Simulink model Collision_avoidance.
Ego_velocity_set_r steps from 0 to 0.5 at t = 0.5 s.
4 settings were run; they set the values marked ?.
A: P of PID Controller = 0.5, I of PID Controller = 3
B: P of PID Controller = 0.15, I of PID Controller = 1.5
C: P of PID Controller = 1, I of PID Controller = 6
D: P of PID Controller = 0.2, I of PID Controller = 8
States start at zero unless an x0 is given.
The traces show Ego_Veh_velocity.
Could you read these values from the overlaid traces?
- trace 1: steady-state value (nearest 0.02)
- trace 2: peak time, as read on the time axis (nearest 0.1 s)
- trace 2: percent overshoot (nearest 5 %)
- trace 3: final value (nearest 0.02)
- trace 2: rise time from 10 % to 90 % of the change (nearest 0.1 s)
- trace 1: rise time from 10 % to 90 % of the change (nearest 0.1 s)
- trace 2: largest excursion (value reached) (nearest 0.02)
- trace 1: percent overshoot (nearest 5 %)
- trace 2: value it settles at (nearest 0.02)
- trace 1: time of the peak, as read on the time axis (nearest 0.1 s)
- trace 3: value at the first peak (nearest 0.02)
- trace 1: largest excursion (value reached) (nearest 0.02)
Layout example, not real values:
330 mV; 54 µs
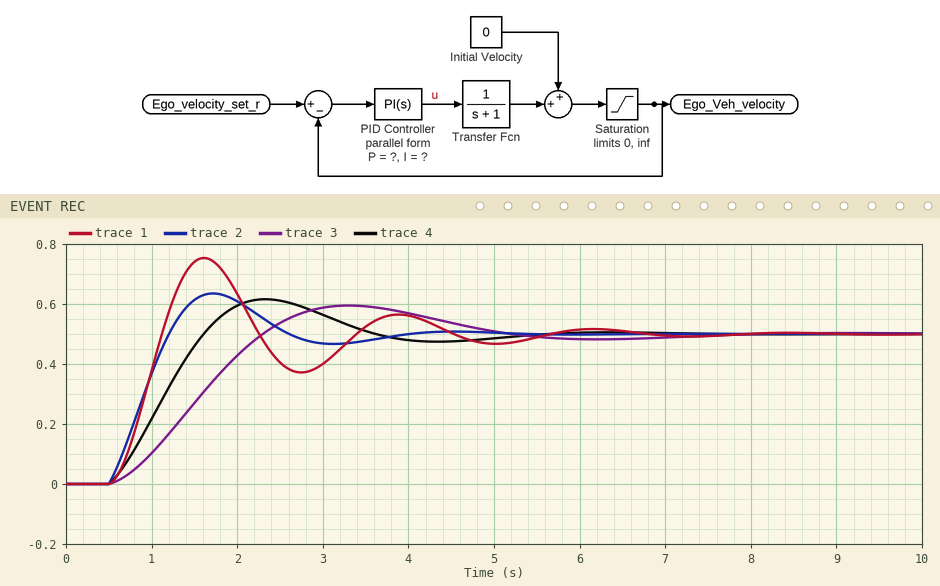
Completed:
0.50; 1.7 s; 25 %; 0.50; 0.5 s; 0.4 s; 0.64; 50 %; 0.50; 1.6 s; 0.60; 0.76
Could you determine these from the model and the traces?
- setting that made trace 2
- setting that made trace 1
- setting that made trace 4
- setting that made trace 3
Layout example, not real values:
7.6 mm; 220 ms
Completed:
C; D; A; B
